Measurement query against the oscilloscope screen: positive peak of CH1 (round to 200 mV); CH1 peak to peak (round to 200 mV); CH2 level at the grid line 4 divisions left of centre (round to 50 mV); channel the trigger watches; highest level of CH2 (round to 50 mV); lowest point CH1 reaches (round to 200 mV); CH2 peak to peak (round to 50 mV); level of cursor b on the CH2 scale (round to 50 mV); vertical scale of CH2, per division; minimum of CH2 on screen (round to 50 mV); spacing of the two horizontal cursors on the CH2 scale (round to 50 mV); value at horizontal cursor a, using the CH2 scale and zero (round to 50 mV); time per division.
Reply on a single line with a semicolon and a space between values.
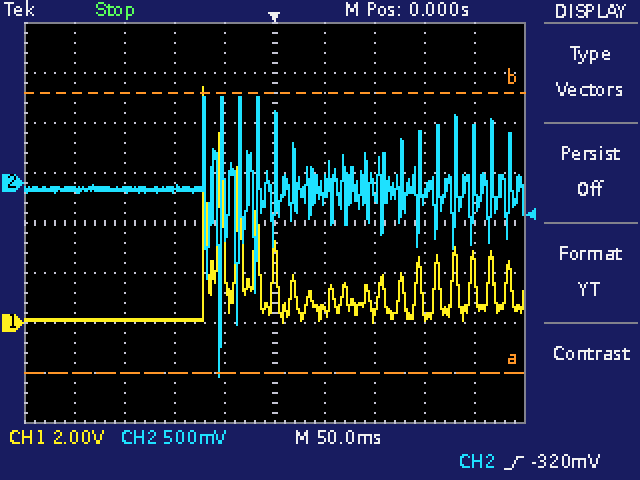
9.4 V; 9.4 V; -50 mV; CH2; 850 mV; 0.0 V; 2.80 V; 900 mV; 500 mV; -1.95 V; 2.80 V; -1.90 V; 50 ms
